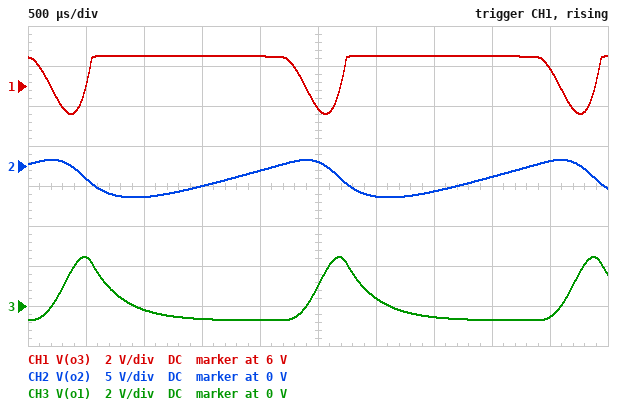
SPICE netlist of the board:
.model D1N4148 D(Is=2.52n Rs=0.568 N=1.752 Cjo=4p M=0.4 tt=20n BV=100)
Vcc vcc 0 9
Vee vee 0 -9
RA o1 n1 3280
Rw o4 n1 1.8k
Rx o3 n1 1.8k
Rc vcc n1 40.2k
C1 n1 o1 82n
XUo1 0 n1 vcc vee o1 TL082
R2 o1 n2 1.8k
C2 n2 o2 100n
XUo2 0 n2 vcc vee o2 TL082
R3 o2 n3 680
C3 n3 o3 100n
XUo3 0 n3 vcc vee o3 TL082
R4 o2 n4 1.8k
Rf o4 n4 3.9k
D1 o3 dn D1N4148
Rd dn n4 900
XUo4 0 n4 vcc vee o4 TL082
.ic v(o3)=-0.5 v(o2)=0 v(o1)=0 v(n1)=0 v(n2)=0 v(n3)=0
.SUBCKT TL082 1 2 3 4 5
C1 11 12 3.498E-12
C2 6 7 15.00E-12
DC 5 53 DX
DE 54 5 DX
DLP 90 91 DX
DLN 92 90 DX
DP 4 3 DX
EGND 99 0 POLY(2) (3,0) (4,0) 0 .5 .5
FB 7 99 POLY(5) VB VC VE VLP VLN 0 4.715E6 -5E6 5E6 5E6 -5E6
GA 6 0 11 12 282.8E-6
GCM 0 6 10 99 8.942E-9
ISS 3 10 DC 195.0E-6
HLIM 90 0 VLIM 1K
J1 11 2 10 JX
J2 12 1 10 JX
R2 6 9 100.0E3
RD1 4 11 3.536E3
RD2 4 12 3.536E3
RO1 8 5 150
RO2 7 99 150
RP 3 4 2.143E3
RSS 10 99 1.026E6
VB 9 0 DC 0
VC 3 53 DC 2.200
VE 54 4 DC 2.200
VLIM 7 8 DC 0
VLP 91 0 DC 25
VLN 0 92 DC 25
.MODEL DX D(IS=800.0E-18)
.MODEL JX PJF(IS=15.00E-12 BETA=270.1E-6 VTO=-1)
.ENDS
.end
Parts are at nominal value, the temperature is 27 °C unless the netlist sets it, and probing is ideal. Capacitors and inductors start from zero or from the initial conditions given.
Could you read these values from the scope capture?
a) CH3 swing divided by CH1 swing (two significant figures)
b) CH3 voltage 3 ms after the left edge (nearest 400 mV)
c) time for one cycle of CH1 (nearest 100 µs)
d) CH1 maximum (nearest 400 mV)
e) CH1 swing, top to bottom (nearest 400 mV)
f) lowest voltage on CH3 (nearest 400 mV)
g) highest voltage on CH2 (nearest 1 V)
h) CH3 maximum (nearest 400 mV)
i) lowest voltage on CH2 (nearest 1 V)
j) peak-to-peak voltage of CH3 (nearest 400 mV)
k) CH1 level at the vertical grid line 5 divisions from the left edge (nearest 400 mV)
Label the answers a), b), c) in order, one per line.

a) 1.1
b) 400 mV
c) 2.2 ms
d) 7.6 V
e) 2.8 V
f) -800 mV
g) 1 V
h) 2.4 V
i) -4 V
j) 3.2 V
k) 4.8 V
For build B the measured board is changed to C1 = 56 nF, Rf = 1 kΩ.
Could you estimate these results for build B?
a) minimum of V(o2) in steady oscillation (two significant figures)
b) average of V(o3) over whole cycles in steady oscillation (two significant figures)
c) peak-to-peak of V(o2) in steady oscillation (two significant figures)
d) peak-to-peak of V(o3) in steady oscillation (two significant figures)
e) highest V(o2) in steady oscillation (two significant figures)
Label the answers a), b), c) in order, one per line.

a) -3.2 V
b) 3.1 V
c) 4.8 V
d) 11 V
e) 1.6 V
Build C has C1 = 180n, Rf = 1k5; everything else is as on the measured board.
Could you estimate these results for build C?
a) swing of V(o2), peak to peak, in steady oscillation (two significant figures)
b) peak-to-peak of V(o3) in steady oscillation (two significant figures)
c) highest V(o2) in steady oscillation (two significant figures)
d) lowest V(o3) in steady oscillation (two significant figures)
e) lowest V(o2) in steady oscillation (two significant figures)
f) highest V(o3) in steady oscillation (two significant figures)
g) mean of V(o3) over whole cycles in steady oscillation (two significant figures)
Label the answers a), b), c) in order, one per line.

a) 3.8 V
b) 4.4 V
c) 870 mV
d) 3.1 V
e) -2.9 V
f) 7.5 V
g) 6.6 V
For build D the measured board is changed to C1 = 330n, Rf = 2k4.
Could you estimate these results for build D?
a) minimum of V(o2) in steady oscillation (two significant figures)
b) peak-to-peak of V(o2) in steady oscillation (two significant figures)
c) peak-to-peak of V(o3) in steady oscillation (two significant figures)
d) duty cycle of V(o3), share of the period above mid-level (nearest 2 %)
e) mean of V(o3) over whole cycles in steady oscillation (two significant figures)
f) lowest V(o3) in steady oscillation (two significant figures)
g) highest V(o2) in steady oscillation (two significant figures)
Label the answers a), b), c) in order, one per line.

a) -5.5 V
b) 6.5 V
c) 6.1 V
d) 86 %
e) 6.7 V
f) 1.4 V
g) 1.0 V
